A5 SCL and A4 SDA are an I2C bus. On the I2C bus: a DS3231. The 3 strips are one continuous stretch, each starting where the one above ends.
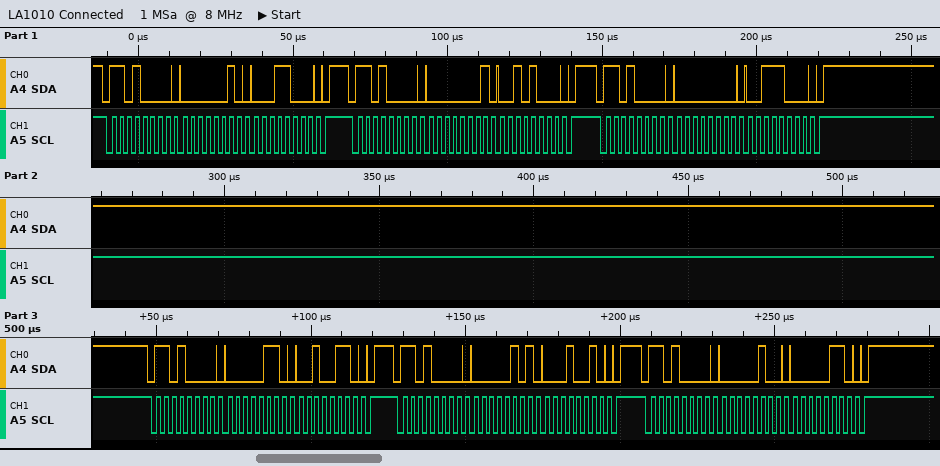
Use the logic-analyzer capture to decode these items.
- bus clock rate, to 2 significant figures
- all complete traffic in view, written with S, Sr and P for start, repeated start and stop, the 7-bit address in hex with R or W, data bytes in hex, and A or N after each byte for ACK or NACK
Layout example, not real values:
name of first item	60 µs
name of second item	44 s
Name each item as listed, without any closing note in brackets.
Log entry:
bus clock rate, to 2 significant figures	400 kHz
all complete traffic in view, written with S, Sr and P for start, repeated start and stop, the 7-bit address in hex with R or W, data bytes in hex, and A or N after each byte for ACK or NACK	S 68W A 02 A 18 A P S 68W A 01 A 28 A P S 68W A 00 A 38 A P S 68W A 06 A 26 A P S 68W A 05 A 12 A P S 68W A 04 A 06 A P
